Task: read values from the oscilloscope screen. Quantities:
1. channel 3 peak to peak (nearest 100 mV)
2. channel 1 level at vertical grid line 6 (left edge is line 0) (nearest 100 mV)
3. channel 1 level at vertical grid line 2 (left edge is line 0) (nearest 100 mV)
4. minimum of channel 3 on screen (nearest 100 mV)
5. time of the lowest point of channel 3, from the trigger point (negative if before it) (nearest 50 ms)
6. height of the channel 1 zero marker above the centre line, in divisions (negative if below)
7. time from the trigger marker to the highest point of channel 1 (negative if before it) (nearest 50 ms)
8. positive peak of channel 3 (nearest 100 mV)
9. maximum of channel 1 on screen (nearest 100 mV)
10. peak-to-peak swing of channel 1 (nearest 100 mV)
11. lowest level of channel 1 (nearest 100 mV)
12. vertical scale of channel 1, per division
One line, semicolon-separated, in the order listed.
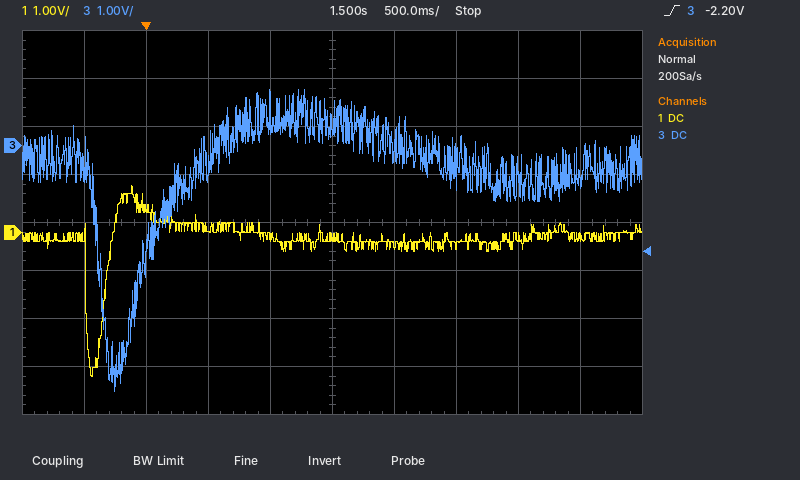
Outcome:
6.3 V; -300 mV; 500 mV; -5.1 V; -250 ms; -0.2 div; -100 ms; 1.2 V; 1.0 V; 4.0 V; -3.0 V; 1 V
